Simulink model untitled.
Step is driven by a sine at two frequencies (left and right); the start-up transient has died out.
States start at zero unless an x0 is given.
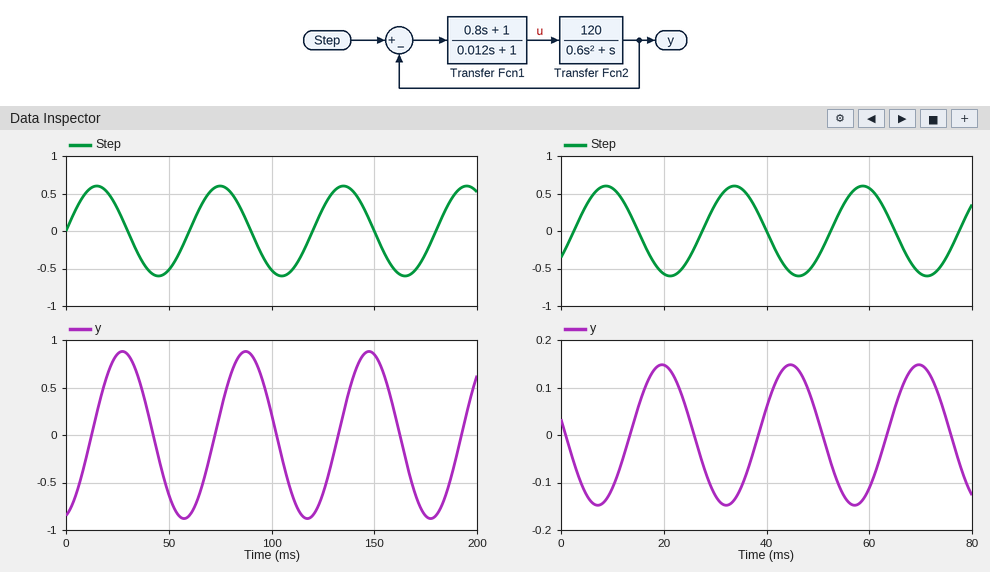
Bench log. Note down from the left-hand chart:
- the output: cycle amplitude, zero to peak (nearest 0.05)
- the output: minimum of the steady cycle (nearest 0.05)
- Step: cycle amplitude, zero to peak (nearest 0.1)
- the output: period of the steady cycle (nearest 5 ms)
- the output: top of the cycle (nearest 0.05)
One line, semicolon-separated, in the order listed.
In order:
0.90; -0.90; 0.6; 60 ms; 0.90
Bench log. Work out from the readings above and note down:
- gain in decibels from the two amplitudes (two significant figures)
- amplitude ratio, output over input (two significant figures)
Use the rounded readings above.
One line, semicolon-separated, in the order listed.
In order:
3.5 dB; 1.5
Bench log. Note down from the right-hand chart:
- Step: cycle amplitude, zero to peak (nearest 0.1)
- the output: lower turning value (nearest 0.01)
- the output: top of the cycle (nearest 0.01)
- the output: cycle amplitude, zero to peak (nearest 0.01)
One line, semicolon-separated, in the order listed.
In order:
0.6; -0.15; 0.15; 0.15
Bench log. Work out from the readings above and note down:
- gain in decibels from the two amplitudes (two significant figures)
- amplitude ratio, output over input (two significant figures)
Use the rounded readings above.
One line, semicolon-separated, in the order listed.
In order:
-12 dB; 0.25
